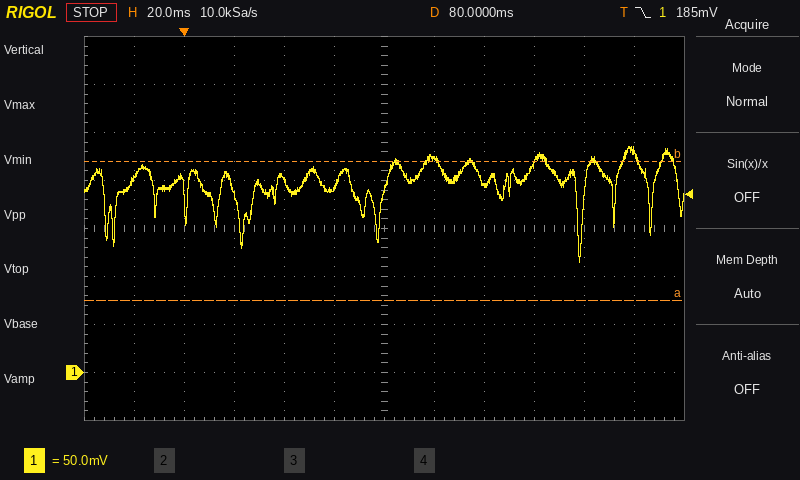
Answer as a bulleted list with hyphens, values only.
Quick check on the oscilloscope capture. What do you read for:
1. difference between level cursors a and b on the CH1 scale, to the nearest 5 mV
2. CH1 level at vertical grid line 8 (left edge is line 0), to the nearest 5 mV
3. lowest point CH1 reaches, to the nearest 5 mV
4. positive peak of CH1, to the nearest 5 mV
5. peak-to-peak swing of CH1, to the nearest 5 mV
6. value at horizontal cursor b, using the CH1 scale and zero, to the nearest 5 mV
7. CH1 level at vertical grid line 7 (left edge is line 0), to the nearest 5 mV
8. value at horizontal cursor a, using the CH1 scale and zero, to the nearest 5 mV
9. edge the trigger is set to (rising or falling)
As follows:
- 145 mV
- 195 mV
- 115 mV
- 235 mV
- 120 mV
- 220 mV
- 220 mV
- 75 mV
- falling
